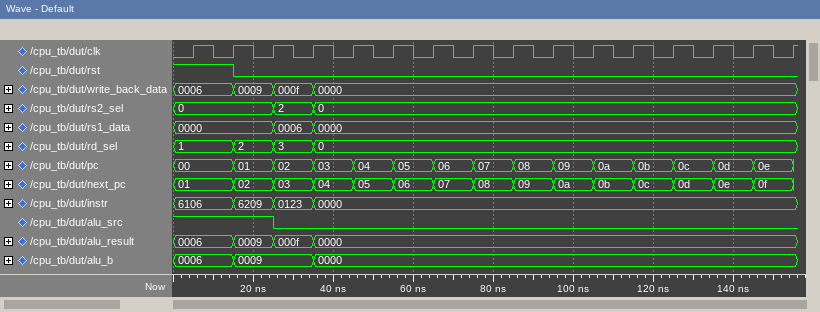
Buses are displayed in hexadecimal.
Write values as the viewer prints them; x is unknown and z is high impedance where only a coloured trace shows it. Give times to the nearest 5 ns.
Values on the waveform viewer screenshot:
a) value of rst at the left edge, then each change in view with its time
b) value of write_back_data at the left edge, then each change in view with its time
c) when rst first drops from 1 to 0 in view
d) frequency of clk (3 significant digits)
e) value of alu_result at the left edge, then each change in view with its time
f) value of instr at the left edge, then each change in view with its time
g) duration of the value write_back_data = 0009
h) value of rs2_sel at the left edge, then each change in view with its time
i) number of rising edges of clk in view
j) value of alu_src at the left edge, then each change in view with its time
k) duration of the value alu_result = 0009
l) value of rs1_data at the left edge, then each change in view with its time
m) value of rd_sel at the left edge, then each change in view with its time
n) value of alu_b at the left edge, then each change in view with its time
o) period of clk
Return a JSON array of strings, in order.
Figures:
["1, 0 at 15 ns", "0006, 0009 at 15 ns, 000f at 25 ns, 0000 at 35 ns", "15 ns", "100 MHz", "0006, 0009 at 15 ns, 000f at 25 ns, 0000 at 35 ns", "6106, 6209 at 15 ns, 0123 at 25 ns, 0000 at 35 ns", "10 ns", "0, 2 at 25 ns, 0 at 35 ns", "16", "1, 0 at 25 ns", "10 ns", "0000, 0006 at 25 ns, 0000 at 35 ns", "1, 2 at 15 ns, 3 at 25 ns, 0 at 35 ns", "0006, 0009 at 15 ns, 0000 at 35 ns", "10 ns"]
